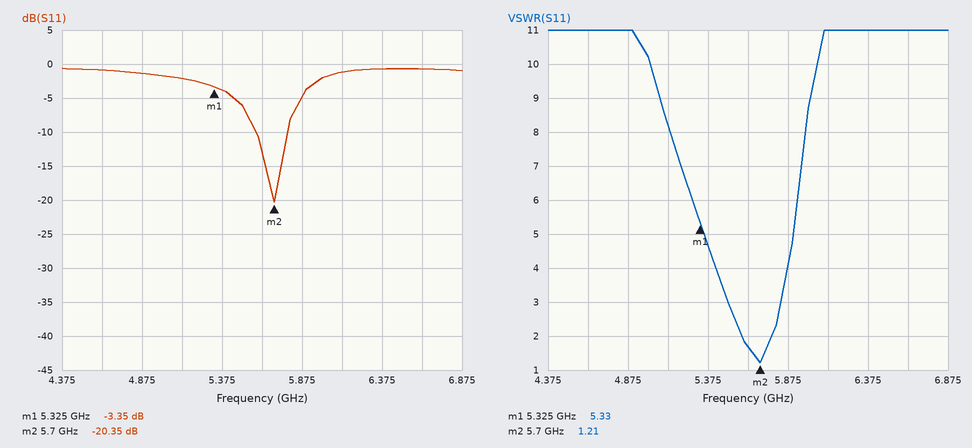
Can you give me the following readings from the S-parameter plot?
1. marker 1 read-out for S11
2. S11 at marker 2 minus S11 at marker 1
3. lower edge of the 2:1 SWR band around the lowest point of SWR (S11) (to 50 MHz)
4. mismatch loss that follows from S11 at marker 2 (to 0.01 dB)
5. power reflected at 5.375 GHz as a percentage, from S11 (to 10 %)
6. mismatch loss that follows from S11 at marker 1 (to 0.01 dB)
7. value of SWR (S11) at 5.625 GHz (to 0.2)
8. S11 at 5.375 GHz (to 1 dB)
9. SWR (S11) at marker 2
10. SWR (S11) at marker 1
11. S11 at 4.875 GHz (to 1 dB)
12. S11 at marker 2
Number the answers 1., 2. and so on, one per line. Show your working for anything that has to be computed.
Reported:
1. -3.35 dB
2. -20.35 − (-3.35) = -17.00 dB
3. 5.60 GHz
4. −10 log10(1 − 10^(-20.35/10)) ≈ 0.04 dB
5. 10^(-4/10) ≈ 40 %
6. −10 log10(1 − 10^(-3.35/10)) ≈ 2.70 dB
7. 1.6
8. -4 dB
9. 1.21
10. 5.33
11. -1 dB
12. -20.35 dB
